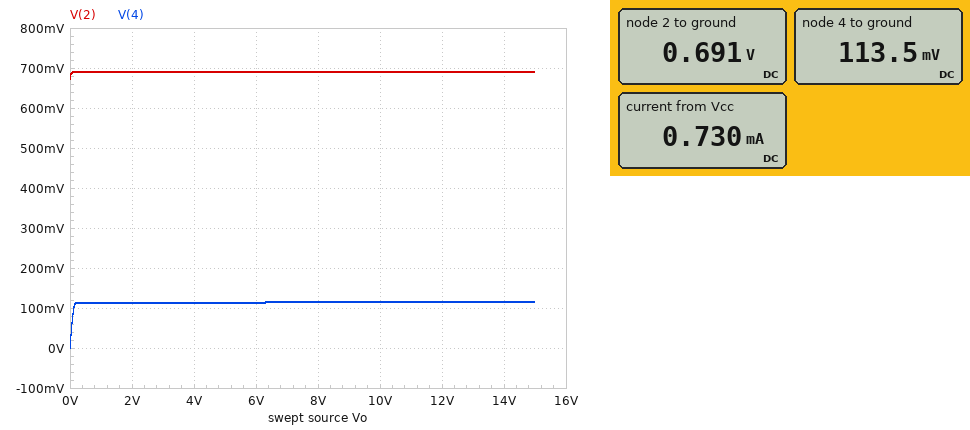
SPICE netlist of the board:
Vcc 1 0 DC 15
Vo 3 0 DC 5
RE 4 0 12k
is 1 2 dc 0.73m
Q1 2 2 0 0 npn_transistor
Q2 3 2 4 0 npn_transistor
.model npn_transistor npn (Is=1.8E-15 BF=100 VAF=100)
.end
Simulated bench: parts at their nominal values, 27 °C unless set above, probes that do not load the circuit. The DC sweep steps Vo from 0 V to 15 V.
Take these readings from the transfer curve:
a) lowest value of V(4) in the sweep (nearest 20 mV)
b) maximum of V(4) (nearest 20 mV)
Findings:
0 V
120 mV
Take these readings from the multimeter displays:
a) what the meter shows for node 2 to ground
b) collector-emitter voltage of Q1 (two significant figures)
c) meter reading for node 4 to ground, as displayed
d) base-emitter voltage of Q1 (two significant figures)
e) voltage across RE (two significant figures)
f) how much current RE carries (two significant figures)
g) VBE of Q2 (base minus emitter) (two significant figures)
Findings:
0.691 V
690 mV
113.5 mV
690 mV
110 mV
9.5 µA
580 mV
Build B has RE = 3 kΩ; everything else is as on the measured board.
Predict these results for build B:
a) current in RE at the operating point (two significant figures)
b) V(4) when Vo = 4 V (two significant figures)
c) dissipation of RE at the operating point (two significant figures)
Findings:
28 µA
85 mV
2.4 µW
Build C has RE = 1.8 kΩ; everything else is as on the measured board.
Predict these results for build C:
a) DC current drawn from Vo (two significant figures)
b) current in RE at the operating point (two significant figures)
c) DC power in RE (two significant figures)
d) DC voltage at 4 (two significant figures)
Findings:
41 µA
42 µA
3.1 µW
75 mV
